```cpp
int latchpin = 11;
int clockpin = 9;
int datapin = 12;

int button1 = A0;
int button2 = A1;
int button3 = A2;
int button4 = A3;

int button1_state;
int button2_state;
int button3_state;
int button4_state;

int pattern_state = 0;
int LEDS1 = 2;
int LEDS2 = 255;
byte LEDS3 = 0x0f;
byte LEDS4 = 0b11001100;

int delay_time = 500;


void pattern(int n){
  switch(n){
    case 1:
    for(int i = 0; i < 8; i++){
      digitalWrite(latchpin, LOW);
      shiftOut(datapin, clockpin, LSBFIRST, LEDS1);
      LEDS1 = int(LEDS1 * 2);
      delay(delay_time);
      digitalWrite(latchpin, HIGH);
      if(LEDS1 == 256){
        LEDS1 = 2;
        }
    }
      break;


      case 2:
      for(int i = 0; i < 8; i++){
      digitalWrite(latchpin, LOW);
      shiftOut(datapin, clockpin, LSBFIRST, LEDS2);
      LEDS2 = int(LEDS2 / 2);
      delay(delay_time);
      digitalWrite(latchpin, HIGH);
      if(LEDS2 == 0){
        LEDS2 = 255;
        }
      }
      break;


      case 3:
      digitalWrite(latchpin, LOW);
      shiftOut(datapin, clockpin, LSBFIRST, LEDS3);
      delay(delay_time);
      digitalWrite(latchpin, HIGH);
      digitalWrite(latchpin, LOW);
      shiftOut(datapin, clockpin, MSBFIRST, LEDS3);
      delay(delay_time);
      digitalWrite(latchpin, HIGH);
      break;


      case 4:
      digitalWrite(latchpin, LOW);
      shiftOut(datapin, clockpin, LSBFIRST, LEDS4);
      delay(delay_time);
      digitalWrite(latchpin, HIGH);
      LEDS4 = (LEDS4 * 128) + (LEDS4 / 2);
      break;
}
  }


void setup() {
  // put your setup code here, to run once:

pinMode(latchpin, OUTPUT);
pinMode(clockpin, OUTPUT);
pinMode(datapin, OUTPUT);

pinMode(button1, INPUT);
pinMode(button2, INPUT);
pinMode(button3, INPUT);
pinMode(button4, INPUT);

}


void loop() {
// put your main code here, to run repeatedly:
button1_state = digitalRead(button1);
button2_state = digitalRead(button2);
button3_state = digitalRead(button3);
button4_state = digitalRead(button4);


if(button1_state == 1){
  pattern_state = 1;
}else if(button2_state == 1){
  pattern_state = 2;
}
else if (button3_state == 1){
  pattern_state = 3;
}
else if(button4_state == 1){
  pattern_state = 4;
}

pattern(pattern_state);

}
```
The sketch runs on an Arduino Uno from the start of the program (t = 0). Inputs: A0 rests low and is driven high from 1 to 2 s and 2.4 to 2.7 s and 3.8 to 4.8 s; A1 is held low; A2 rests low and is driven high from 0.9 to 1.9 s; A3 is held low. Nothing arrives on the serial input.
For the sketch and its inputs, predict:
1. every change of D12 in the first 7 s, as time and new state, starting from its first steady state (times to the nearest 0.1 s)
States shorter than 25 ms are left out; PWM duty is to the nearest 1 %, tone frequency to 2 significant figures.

0 s low; 1.4 s high; 1.9 s low; 4.9 s high; 5.4 s low
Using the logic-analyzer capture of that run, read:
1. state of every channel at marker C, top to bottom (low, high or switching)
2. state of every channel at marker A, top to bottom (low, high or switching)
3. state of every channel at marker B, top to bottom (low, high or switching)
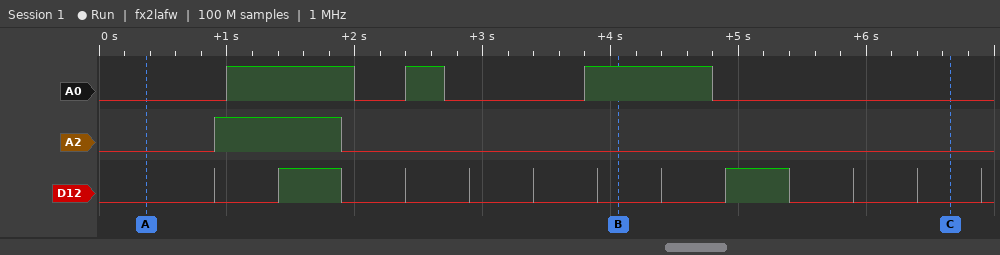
A0 low, A2 low, D12 low
A0 low, A2 low, D12 low
A0 high, A2 low, D12 low
